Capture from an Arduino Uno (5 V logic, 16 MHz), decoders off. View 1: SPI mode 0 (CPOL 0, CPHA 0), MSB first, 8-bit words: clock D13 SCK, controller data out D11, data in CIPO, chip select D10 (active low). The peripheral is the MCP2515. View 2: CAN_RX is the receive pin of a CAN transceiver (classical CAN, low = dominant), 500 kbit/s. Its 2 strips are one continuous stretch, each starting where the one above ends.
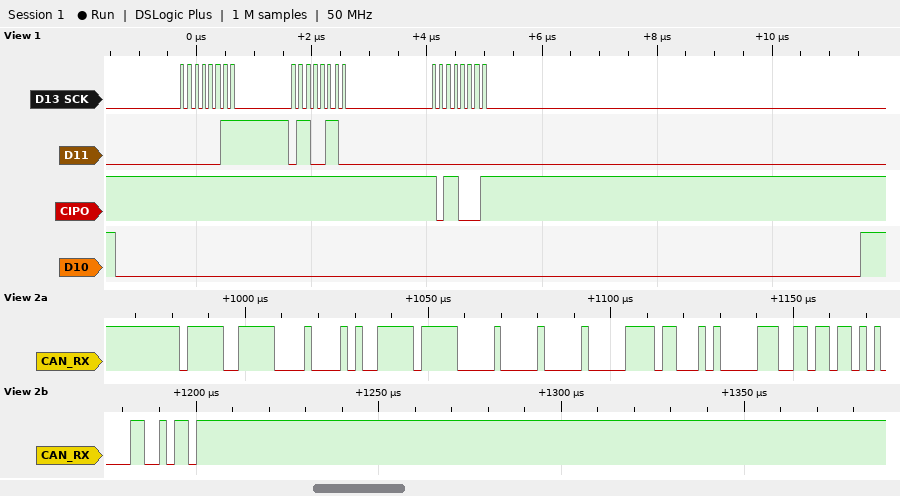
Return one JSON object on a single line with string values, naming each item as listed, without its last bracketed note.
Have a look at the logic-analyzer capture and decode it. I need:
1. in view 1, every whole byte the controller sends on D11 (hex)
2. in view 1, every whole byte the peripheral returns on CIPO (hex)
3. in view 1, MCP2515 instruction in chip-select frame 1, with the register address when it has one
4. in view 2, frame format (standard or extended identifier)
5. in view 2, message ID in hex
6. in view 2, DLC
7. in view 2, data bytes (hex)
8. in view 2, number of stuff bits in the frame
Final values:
{"in view 1, every whole byte the controller sends on D11": "03 66 00", "in view 1, every whole byte the peripheral returns on CIPO": "FF FF B1", "in view 1, MCP2515 instruction in chip-select frame 1, with the register address when it has one": "READ 0x66", "in view 2, frame format": "standard", "in view 2, message ID in hex": "0x7DF", "in view 2, DLC": "8", "in view 2, data bytes": "53 FF 00 00 1D 8A 0C DB", "in view 2, number of stuff bits in the frame": "9"}
